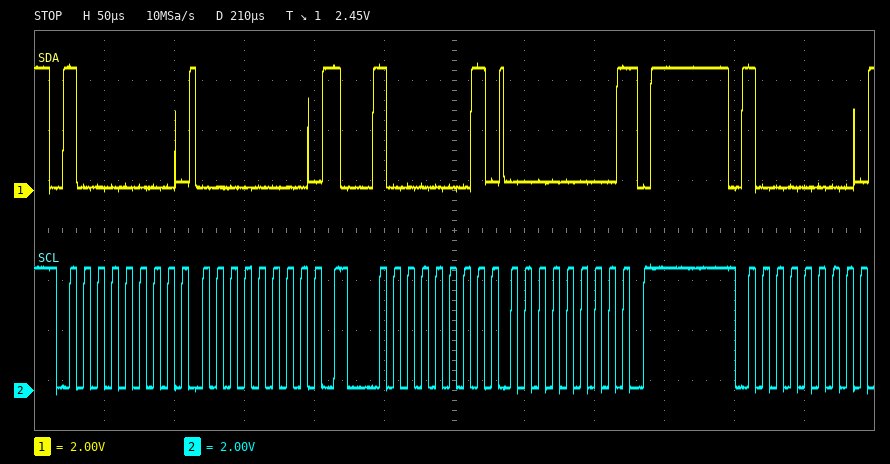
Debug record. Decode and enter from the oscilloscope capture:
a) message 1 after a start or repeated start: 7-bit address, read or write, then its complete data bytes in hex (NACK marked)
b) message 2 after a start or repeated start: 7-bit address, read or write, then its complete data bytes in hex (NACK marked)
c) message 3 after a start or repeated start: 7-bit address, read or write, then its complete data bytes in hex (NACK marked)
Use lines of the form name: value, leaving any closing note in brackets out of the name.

message 1 after a start or repeated start: 7-bit address, read or write, then its complete data bytes in hex: 0x40 write: 00
message 2 after a start or repeated start: 7-bit address, read or write, then its complete data bytes in hex: 0x40 read: 00 NACK
message 3 after a start or repeated start: 7-bit address, read or write, then its complete data bytes in hex: 0x40 write
